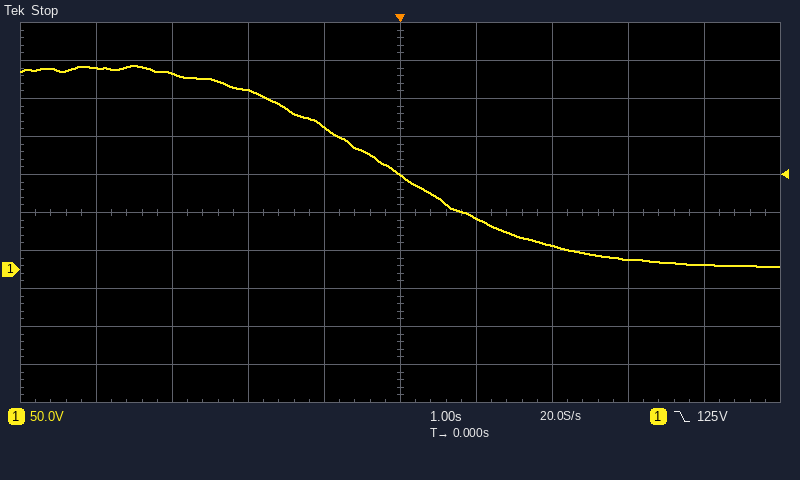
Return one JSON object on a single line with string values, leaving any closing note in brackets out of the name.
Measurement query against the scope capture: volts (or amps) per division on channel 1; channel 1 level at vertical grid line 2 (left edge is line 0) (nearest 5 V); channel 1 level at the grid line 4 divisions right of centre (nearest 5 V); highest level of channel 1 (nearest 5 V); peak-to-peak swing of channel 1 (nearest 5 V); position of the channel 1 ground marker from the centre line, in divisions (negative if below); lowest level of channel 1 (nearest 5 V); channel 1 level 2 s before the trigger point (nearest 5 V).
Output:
{"volts (or amps) per division on channel 1": "50 V", "channel 1 level at vertical grid line 2 (left edge is line 0)": "260 V", "channel 1 level at the grid line 4 divisions right of centre": "5 V", "highest level of channel 1": "270 V", "peak-to-peak swing of channel 1": "265 V", "position of the channel 1 ground marker from the centre line, in divisions": "-1.5 div", "lowest level of channel 1": "5 V", "channel 1 level 2 s before the trigger point": "235 V"}
